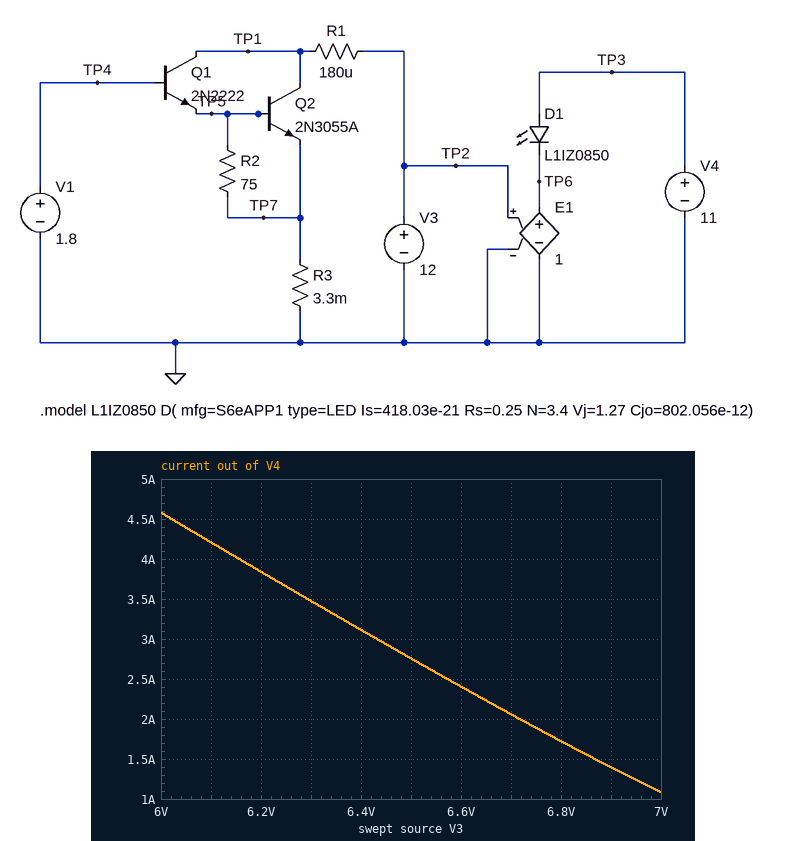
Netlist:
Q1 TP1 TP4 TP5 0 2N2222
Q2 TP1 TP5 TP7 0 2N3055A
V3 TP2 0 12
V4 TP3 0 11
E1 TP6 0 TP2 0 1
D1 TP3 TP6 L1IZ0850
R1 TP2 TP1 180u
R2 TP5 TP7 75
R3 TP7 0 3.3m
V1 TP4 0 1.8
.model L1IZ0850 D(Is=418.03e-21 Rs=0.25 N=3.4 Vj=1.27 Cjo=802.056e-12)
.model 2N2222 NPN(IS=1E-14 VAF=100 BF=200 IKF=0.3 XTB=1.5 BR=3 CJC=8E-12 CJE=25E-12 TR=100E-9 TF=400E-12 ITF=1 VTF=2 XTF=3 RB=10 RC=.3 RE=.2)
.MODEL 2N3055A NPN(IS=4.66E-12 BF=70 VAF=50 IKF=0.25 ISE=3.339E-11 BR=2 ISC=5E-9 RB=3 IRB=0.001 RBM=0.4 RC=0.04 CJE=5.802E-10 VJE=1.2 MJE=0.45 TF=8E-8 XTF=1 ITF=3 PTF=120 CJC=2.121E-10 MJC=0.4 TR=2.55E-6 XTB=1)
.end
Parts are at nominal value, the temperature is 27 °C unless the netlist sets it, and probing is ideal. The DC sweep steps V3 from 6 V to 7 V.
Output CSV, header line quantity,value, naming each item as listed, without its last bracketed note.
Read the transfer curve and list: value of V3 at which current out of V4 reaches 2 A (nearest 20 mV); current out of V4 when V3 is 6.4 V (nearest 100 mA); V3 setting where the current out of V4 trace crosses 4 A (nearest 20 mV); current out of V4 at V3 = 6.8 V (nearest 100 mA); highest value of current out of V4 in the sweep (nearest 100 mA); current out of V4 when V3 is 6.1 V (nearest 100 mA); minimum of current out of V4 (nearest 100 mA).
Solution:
quantity,value
value of V3 at which current out of V4 reaches 2 A,6.72 V
current out of V4 when V3 is 6.4 V,3.1 A
V3 setting where the current out of V4 trace crosses 4 A,6.16 V
current out of V4 at V3 = 6.8 V,1.7 A
highest value of current out of V4 in the sweep,4.6 A
current out of V4 when V3 is 6.1 V,4.2 A
minimum of current out of V4,1.1 A
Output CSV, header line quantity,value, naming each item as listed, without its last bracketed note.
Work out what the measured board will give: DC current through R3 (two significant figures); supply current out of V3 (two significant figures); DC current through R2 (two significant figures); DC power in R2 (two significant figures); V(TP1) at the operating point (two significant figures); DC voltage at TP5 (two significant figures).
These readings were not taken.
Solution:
quantity,value
DC current through R3,2.8 A
supply current out of V3,2.8 A
DC current through R2,12 mA
DC power in R2,11 mW
V(TP1) at the operating point,12 V
DC voltage at TP5,900 mV
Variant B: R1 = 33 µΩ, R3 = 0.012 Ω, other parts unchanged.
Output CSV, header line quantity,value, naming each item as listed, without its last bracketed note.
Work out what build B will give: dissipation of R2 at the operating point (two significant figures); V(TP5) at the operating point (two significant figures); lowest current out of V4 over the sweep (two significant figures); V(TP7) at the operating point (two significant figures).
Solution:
quantity,value
dissipation of R2 at the operating point,10 mW
V(TP5) at the operating point,910 mV
lowest current out of V4 over the sweep,1.1 A
V(TP7) at the operating point,32 mV
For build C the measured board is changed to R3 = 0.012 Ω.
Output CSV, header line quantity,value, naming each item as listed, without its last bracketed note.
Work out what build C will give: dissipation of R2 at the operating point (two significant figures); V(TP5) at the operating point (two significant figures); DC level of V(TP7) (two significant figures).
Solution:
quantity,value
dissipation of R2 at the operating point,10 mW
V(TP5) at the operating point,910 mV
DC level of V(TP7),32 mV
